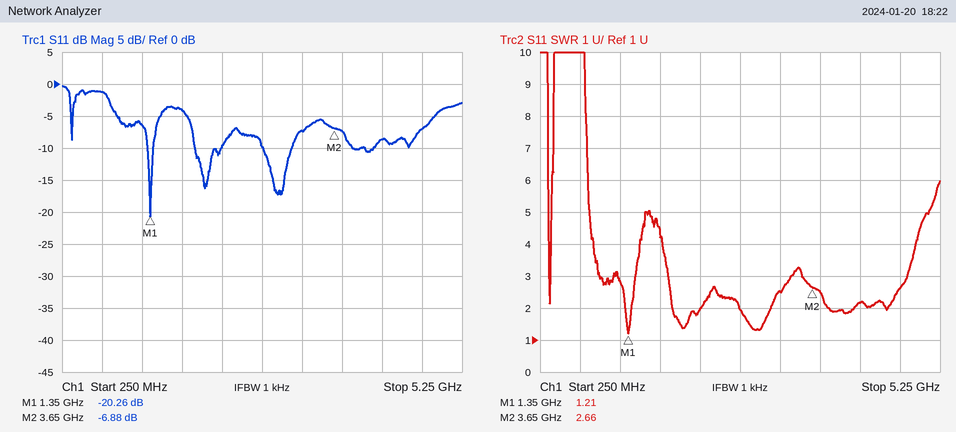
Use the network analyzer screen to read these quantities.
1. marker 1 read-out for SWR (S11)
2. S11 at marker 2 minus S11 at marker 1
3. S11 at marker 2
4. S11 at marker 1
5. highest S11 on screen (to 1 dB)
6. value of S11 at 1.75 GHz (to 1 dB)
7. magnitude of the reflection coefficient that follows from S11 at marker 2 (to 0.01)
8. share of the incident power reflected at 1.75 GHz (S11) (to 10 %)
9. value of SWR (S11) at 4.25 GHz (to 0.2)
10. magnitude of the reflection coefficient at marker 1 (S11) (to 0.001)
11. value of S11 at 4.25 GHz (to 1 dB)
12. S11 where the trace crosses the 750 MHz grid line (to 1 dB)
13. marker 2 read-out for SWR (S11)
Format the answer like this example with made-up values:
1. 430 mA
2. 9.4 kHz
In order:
1. 1.21
2. 13.38 dB
3. -6.88 dB
4. -20.26 dB
5. 0 dB
6. -4 dB
7. 0.45
8. 40 %
9. 2.2
10. 0.097
11. -9 dB
12. -1 dB
13. 2.66
